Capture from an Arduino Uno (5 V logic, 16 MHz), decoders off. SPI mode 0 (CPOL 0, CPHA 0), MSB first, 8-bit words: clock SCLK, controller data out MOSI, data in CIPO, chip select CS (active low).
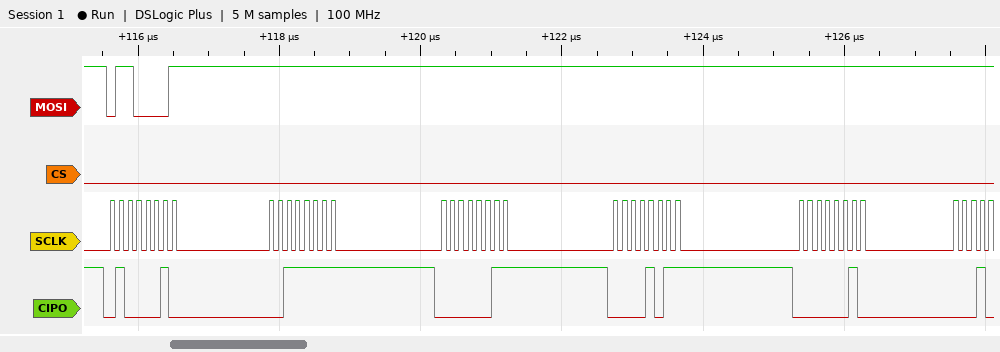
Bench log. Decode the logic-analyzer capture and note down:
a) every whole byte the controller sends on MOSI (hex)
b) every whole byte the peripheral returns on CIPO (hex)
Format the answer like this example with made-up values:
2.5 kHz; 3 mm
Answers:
61 FF FF FF FF; 42 3F 03 0B 02
